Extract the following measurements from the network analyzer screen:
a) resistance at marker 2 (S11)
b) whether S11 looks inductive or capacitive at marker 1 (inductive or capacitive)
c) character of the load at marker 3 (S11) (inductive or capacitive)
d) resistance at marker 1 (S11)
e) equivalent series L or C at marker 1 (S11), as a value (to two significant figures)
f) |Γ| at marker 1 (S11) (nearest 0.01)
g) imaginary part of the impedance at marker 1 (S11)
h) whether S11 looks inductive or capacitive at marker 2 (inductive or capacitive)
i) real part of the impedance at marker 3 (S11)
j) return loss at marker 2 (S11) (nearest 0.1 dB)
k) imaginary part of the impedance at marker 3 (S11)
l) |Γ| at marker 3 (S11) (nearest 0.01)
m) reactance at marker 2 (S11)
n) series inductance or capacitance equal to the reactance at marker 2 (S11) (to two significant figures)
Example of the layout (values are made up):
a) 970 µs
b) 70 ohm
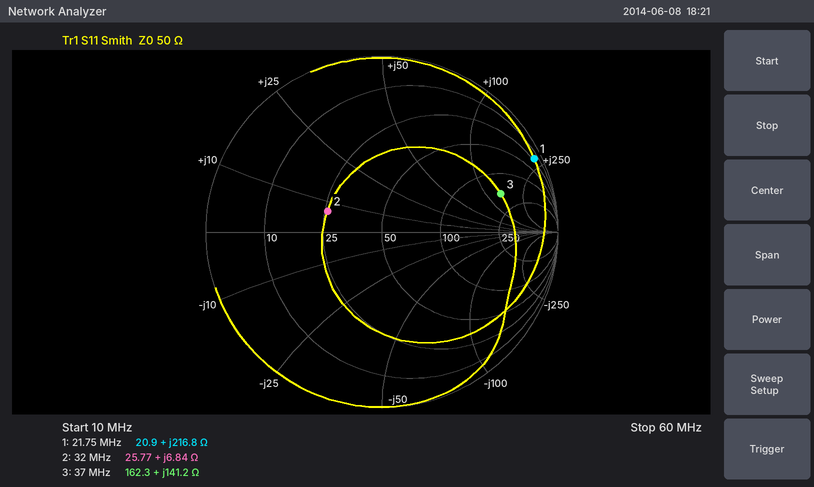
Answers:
a) 25.77 Ω
b) inductive
c) inductive
d) 20.9 Ω
e) 1.6 µH
f) 0.96
g) +216.8 Ω
h) inductive
i) 162.3 Ω
j) 9.6 dB
k) +141.2 Ω
l) 0.71
m) +6.84 Ω
n) 34 nH
